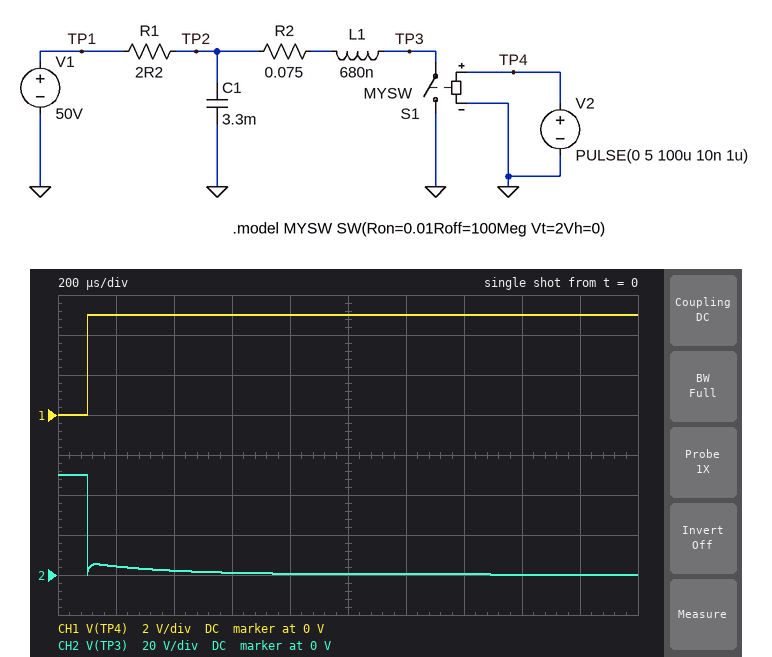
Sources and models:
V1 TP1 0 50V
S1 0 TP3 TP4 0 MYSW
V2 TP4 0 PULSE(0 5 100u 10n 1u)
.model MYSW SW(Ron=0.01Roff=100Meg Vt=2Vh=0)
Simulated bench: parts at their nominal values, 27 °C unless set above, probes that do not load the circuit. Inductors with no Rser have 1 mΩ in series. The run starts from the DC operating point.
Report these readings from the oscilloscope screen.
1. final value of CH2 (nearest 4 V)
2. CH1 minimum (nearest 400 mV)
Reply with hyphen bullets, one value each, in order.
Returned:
- 0 V
- 0 V
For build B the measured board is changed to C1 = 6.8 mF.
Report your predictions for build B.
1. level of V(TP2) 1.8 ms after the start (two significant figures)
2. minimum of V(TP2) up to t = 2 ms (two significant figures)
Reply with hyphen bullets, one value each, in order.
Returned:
- 4.2 V
- 3.5 V
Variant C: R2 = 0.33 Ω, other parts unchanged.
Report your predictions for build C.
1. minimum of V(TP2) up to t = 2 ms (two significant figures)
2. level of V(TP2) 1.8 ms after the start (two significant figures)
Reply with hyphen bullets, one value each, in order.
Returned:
- 13 V
- 14 V
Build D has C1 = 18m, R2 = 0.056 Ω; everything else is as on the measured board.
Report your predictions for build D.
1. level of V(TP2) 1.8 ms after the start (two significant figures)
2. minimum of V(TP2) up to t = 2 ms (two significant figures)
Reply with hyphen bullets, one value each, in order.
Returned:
- 13 V
- 11 V
